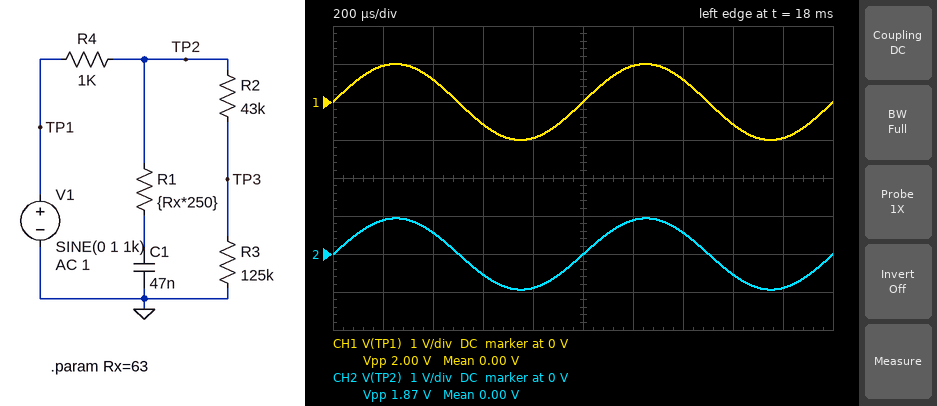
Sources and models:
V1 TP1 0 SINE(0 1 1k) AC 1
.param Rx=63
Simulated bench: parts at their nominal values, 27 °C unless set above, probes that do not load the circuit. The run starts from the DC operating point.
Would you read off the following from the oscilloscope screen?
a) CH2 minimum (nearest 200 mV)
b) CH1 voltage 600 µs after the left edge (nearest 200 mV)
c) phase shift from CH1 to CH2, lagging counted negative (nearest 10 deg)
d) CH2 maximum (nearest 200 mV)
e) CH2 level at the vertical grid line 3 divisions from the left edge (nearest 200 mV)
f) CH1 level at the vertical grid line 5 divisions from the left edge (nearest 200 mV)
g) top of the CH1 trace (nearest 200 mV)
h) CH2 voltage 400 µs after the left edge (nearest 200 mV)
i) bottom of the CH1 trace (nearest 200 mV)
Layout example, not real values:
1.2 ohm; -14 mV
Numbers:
-1.0 V; -600 mV; 0 deg; 1.0 V; -600 mV; 0 V; 1.0 V; 600 mV; -1.0 V
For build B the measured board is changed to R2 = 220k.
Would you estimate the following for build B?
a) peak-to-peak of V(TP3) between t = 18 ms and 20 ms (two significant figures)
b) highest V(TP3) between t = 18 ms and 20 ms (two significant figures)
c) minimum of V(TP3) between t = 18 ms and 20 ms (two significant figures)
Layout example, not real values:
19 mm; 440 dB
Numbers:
680 mV; 340 mV; -340 mV
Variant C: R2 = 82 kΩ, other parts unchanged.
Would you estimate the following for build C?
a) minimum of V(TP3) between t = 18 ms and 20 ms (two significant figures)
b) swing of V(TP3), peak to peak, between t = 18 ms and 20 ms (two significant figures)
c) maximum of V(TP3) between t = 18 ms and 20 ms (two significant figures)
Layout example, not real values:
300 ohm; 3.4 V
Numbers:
-570 mV; 1.1 V; 570 mV
